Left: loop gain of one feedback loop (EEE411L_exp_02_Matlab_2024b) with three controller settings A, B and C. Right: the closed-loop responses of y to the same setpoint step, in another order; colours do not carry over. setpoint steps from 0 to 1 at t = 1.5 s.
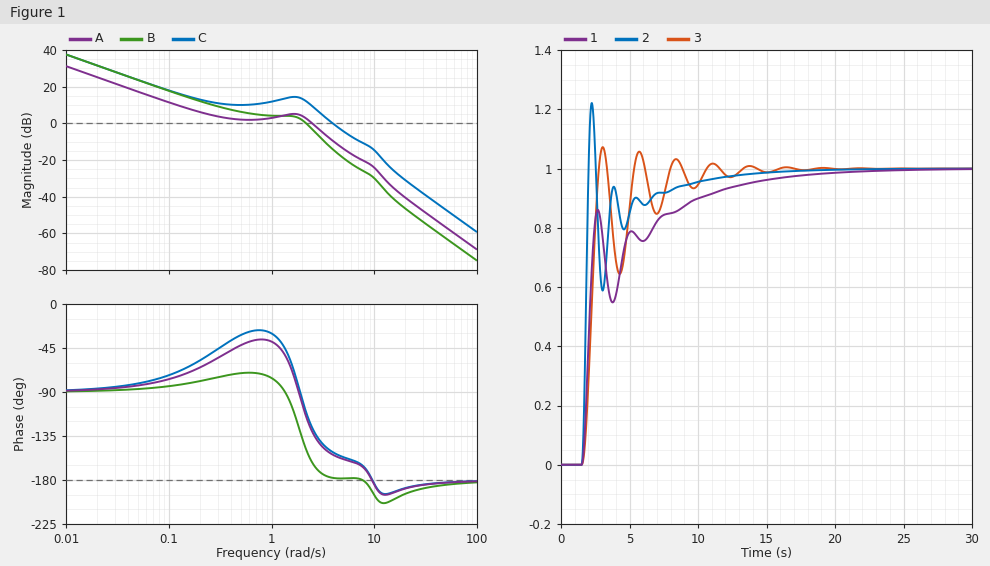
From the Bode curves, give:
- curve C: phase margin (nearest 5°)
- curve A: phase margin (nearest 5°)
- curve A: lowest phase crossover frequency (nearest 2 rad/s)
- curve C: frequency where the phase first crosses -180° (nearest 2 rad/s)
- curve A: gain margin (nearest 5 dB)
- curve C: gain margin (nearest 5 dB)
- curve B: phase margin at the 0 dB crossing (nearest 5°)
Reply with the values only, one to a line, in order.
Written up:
30°
50°
10 rad/s
10 rad/s
25 dB
15 dB
30°
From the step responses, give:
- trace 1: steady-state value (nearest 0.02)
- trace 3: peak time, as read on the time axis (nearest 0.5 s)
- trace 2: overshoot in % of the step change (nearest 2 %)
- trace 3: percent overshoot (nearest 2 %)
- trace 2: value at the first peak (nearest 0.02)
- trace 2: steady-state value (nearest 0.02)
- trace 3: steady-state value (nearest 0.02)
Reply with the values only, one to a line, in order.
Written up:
1.00
3.0 s
22 %
8 %
1.22
1.00
1.00
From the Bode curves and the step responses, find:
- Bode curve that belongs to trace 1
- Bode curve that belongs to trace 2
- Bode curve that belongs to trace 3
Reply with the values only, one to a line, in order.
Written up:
A
C
B
